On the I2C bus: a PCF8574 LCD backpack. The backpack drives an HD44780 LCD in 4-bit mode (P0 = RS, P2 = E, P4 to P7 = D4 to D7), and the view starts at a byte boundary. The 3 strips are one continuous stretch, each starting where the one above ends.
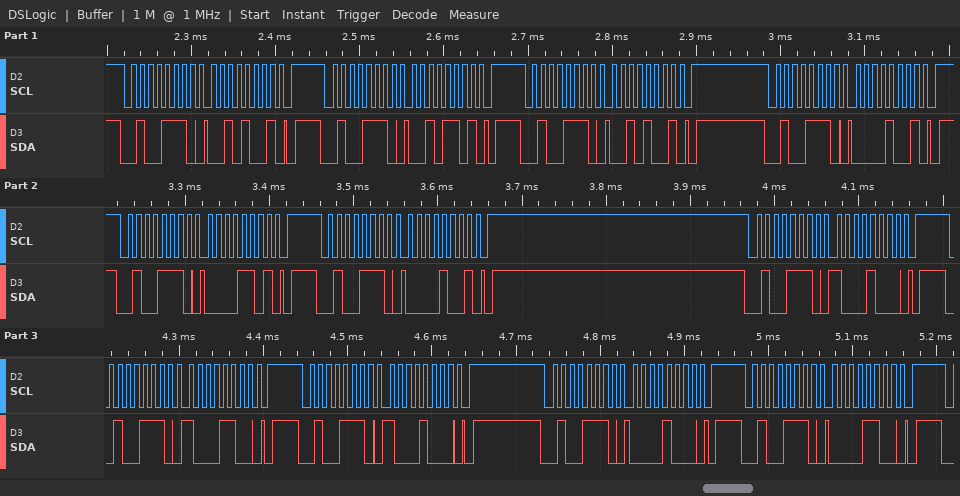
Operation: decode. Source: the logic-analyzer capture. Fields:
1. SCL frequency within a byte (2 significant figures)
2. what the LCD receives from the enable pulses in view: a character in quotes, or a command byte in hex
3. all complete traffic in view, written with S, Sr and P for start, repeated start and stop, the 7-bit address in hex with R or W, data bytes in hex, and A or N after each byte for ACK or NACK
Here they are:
100 kHz
' '
S 27W A 29 A P S 27W A 2D A P S 27W A 29 A P S 27W A 09 A P S 27W A 0D A P S 27W A 09 A P S 27W A 88 A P S 27W A 8C A P S 27W A 88 A P S 27W A 08 A P S 27W A 0C A P
